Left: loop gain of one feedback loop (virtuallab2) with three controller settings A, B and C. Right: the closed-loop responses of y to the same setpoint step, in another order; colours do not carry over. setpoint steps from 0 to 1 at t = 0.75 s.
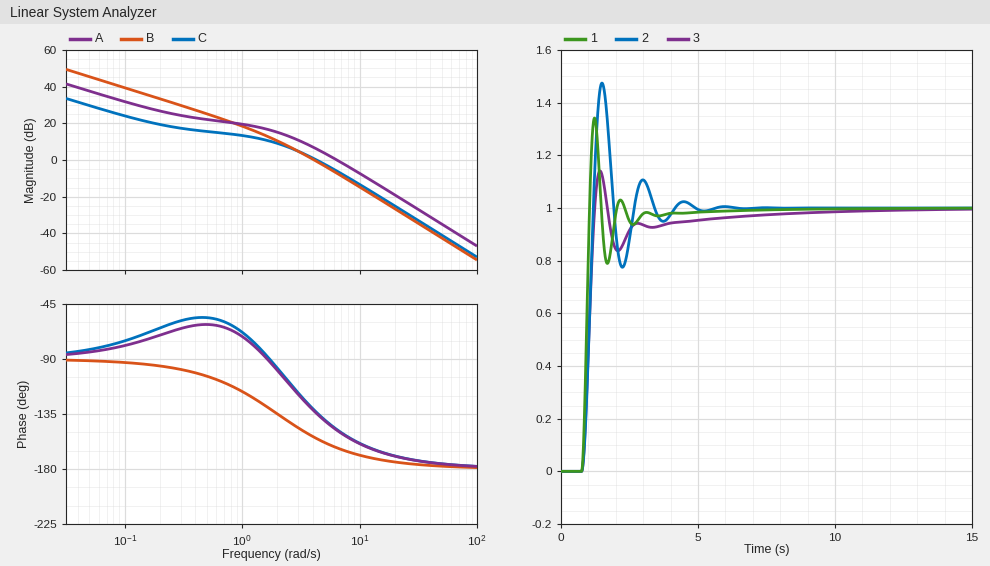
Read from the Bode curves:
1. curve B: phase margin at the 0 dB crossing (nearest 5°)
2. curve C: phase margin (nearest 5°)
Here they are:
25°
45°
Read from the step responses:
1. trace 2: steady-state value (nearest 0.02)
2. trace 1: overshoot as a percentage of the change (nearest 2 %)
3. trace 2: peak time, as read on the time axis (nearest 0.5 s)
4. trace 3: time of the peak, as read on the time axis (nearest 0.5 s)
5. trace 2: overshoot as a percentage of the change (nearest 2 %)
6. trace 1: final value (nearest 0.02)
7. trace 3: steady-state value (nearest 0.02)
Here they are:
1.00
34 %
1.5 s
1.5 s
48 %
1.00
1.00
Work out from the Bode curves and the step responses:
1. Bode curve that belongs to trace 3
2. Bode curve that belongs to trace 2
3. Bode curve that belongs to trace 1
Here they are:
C
B
A
